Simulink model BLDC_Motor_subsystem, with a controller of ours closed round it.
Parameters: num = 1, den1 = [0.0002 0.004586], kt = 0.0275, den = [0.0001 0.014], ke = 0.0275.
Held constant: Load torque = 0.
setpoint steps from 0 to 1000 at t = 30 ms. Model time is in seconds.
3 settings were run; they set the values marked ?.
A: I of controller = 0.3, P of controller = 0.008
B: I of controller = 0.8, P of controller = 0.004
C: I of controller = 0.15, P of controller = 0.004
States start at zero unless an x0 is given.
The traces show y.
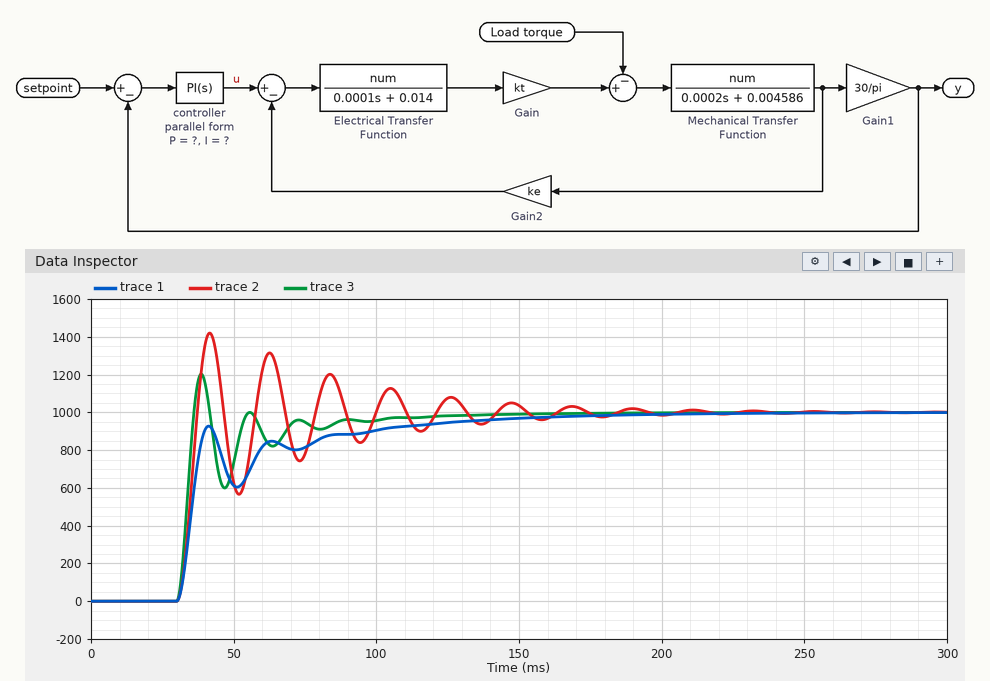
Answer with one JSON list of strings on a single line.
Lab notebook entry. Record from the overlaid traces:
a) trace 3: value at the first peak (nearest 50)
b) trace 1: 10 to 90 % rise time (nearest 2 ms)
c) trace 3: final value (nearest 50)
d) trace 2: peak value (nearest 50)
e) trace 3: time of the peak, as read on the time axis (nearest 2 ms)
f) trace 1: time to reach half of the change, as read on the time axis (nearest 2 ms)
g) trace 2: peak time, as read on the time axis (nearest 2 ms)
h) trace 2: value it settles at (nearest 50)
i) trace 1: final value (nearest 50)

["1200", "8 ms", "1000", "1400", "38 ms", "36 ms", "42 ms", "1000", "1000"]
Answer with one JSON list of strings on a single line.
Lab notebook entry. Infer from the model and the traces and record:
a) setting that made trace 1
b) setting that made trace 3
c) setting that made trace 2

["C", "A", "B"]
